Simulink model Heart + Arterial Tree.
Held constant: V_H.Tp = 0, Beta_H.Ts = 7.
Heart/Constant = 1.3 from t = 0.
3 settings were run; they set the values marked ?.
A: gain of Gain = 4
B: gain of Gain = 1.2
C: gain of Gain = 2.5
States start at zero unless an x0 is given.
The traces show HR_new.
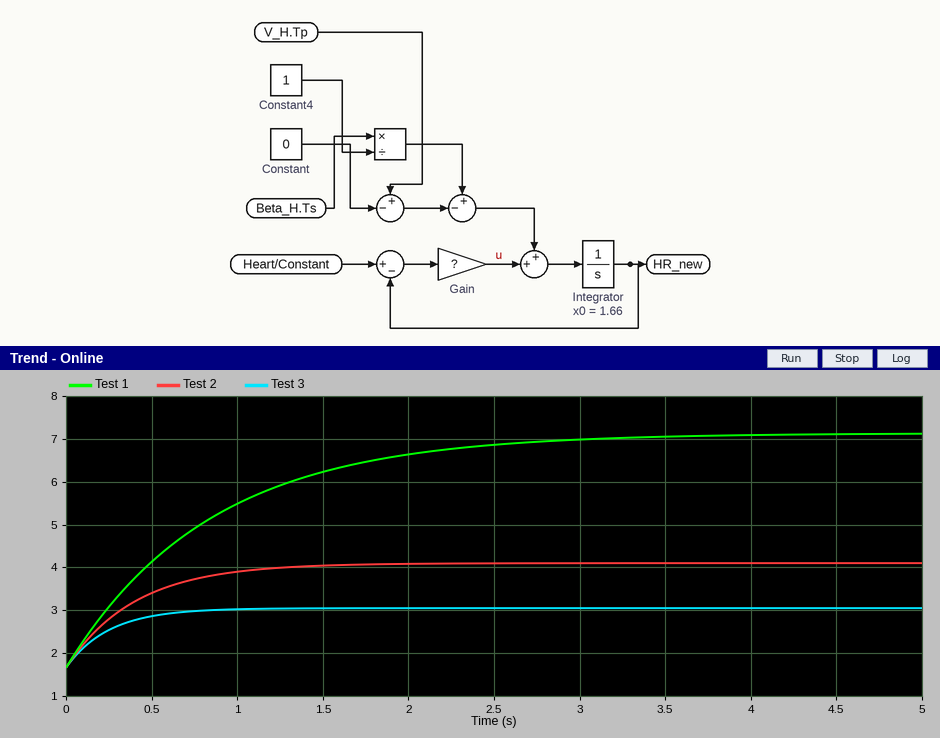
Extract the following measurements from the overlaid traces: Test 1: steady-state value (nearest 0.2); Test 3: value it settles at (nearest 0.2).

7.2
3.0
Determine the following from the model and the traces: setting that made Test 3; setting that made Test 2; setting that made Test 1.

A
C
B
